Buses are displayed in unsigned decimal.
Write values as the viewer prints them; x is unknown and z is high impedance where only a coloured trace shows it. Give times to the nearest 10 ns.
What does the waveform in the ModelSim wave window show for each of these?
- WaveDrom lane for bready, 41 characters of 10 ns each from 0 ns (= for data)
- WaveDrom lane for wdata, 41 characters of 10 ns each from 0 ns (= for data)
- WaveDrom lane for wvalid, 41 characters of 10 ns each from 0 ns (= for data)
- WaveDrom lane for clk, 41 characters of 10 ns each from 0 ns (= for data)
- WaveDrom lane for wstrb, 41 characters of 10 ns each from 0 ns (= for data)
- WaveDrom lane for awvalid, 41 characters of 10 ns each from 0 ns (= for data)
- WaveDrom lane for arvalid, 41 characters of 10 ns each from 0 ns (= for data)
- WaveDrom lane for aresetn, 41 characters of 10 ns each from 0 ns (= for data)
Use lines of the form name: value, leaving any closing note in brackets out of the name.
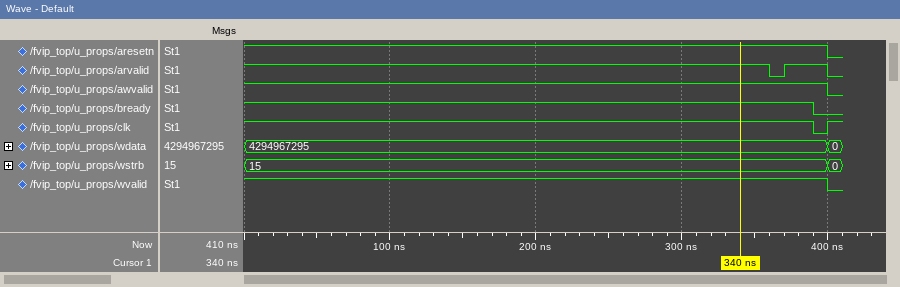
WaveDrom lane for bready, 41 characters of 10 ns each from 0 ns: {name: 'bready', wave: '1......................................0.'}
WaveDrom lane for wdata, 41 characters of 10 ns each from 0 ns: {name: 'wdata', wave: '=.......................................=', data: '4294967295 0'}
WaveDrom lane for wvalid, 41 characters of 10 ns each from 0 ns: {name: 'wvalid', wave: '1.......................................0'}
WaveDrom lane for clk, 41 characters of 10 ns each from 0 ns: {name: 'clk', wave: '1......................................01'}
WaveDrom lane for wstrb, 41 characters of 10 ns each from 0 ns: {name: 'wstrb', wave: '=.......................................=', data: '15 0'}
WaveDrom lane for awvalid, 41 characters of 10 ns each from 0 ns: {name: 'awvalid', wave: '1.......................................0'}
WaveDrom lane for arvalid, 41 characters of 10 ns each from 0 ns: {name: 'arvalid', wave: '1...................................01..0'}
WaveDrom lane for aresetn, 41 characters of 10 ns each from 0 ns: {name: 'aresetn', wave: '1.......................................0'}
